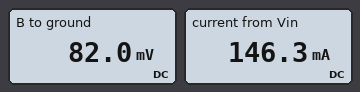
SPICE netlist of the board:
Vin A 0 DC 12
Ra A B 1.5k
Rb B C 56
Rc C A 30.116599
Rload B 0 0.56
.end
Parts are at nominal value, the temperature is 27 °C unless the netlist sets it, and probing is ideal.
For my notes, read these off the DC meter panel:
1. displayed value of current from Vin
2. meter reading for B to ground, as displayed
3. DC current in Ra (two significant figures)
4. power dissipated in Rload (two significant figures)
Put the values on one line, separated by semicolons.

146.3 mA; 82.0 mV; 7.9 mA; 12 mW
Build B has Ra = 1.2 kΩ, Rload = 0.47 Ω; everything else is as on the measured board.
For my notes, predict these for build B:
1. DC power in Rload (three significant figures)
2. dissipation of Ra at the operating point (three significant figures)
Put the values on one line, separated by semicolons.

10.4 mW; 119 mW
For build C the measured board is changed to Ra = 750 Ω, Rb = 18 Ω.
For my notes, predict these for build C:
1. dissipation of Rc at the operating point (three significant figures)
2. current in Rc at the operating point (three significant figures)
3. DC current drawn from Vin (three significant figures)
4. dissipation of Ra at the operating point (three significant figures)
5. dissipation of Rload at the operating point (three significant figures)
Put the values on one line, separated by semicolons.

1.83 W; 246 mA; 262 mA; 187 mW; 38.5 mW
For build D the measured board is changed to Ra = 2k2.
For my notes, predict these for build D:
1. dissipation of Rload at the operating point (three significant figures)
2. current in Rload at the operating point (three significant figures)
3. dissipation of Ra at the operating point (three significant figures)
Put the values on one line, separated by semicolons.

11.6 mW; 144 mA; 64.6 mW
